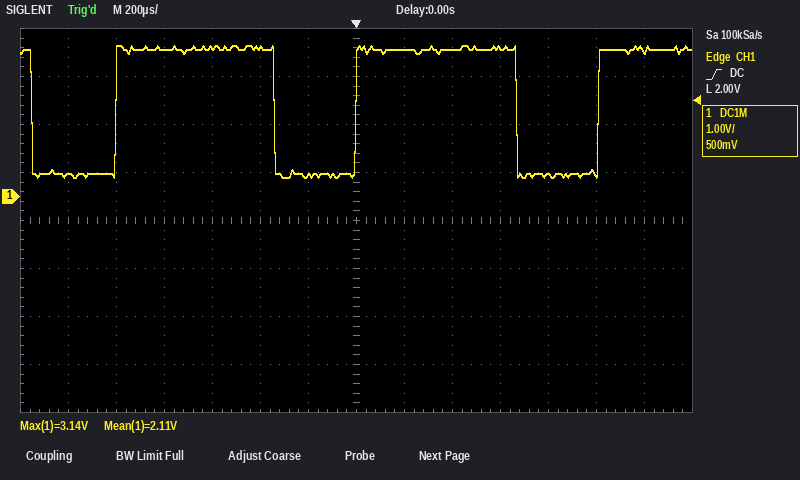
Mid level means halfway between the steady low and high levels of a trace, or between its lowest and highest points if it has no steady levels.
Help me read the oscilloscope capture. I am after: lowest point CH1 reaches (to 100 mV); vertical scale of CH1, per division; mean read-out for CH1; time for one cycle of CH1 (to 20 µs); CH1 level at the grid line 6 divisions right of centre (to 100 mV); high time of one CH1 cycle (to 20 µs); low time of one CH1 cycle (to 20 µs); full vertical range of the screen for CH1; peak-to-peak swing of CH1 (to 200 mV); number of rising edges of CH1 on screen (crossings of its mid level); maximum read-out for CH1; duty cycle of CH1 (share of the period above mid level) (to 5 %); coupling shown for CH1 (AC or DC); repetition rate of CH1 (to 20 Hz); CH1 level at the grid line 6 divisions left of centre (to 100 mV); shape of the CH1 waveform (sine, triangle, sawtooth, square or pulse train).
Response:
400 mV
1 V
2.11 V
1.00 ms
3.0 V
660 µs
340 µs
8 V
2.8 V
3
3.14 V
65 %
DC
1.00 kHz
500 mV
pulse train
